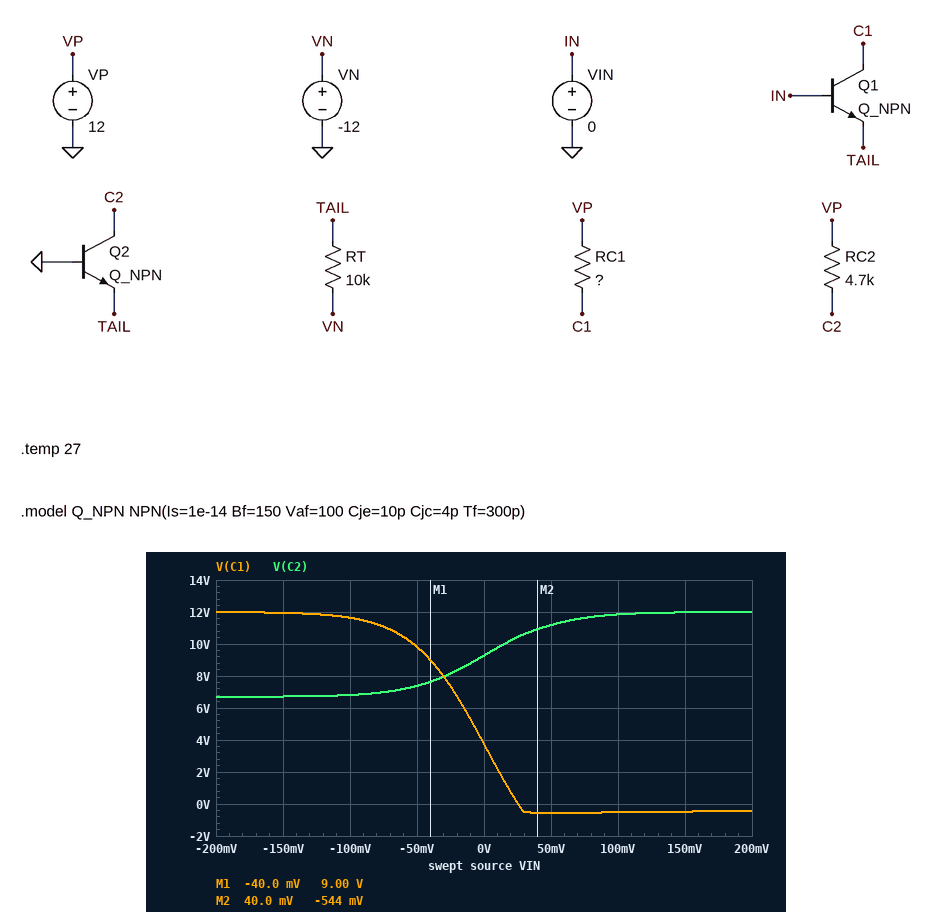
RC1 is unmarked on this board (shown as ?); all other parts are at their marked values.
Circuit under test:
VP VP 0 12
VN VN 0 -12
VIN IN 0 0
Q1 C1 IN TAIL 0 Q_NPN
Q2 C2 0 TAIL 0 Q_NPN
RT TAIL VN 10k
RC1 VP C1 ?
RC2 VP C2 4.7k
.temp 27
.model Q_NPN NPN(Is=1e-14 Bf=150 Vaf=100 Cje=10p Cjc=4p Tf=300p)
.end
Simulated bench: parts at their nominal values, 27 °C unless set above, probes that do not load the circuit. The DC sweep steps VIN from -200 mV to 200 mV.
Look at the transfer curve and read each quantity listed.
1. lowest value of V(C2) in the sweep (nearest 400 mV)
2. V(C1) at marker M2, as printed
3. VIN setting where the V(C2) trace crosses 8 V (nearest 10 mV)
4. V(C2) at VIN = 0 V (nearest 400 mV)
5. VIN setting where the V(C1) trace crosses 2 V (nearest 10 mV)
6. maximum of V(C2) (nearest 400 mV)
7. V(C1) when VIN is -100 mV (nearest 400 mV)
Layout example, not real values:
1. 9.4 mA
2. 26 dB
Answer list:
1. 6.8 V
2. -544 mV
3. -30 mV
4. 9.2 V
5. 10 mV
6. 12.0 V
7. 11.6 V
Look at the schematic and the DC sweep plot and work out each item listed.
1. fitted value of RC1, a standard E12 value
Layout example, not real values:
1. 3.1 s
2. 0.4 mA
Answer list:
1. 15 kΩ
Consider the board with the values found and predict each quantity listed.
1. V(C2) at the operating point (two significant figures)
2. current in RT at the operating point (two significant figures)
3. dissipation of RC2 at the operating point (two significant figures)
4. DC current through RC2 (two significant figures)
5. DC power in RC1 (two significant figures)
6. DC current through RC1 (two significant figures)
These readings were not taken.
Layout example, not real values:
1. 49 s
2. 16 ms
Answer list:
1. 9.3 V
2. 1.1 mA
3. 1.6 mW
4. 580 µA
5. 4.5 mW
6. 550 µA
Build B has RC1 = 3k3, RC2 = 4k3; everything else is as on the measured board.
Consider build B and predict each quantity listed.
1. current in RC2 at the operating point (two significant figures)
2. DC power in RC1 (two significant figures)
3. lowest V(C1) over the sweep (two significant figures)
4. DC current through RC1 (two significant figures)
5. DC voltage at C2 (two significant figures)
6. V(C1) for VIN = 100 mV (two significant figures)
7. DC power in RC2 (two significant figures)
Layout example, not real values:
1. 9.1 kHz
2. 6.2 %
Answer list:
1. 560 µA
2. 1.1 mW
3. 8.2 V
4. 570 µA
5. 9.6 V
6. 8.3 V
7. 1.4 mW
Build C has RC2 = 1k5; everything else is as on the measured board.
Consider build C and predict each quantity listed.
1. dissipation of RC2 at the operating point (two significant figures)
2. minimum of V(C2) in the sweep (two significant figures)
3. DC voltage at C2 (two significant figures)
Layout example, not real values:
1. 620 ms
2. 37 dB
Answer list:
1. 510 µW
2. 10 V
3. 11 V
